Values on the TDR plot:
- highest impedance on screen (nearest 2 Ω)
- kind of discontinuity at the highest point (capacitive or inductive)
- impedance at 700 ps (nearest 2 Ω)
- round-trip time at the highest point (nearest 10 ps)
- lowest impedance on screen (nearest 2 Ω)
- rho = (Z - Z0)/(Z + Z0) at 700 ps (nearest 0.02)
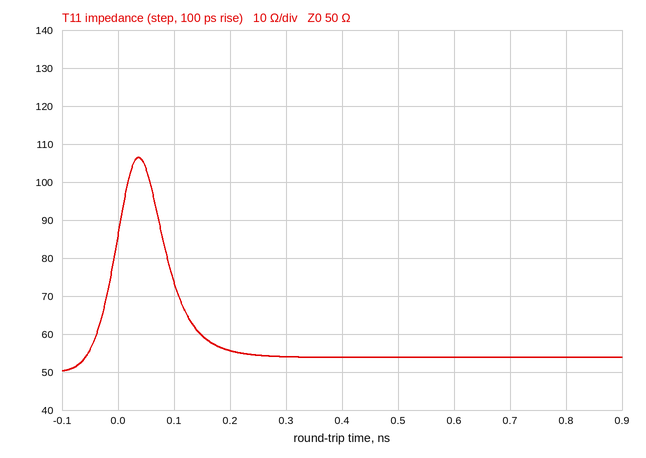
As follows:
106 Ω
inductive
54 Ω
40 ps
50 Ω
+0.04
